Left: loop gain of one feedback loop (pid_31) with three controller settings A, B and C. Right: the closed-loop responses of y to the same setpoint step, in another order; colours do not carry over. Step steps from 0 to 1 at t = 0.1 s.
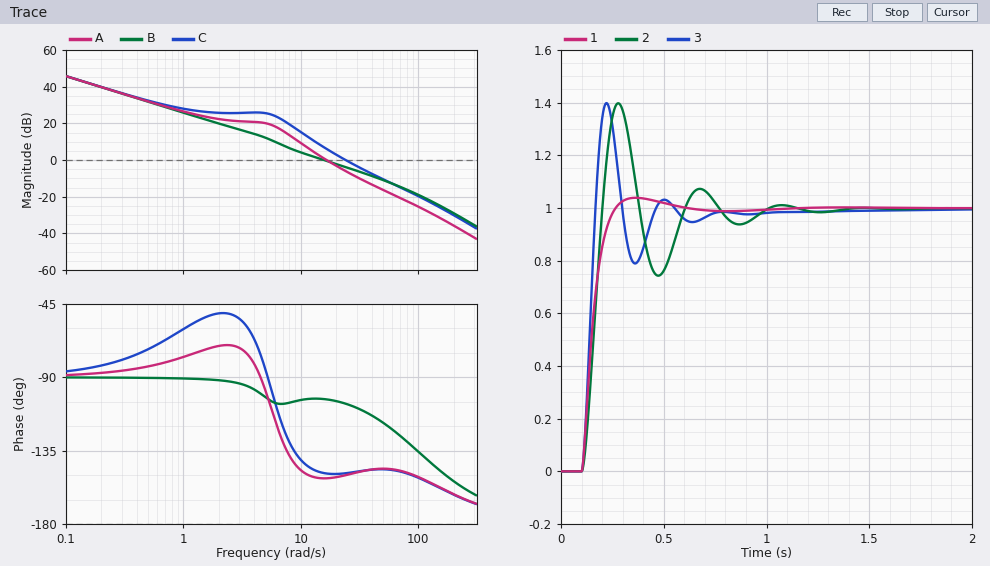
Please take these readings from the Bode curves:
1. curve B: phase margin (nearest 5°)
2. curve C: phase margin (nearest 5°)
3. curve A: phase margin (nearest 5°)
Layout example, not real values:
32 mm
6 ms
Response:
75°
30°
30°
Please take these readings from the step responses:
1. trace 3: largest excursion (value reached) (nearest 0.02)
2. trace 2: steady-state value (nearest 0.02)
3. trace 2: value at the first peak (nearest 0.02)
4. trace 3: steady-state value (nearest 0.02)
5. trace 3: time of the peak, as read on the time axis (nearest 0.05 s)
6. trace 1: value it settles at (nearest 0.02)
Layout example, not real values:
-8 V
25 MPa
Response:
1.40
1.00
1.40
1.00
0.20 s
1.00
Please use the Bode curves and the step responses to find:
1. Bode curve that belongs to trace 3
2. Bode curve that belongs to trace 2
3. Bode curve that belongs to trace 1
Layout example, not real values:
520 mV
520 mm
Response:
C
A
B
